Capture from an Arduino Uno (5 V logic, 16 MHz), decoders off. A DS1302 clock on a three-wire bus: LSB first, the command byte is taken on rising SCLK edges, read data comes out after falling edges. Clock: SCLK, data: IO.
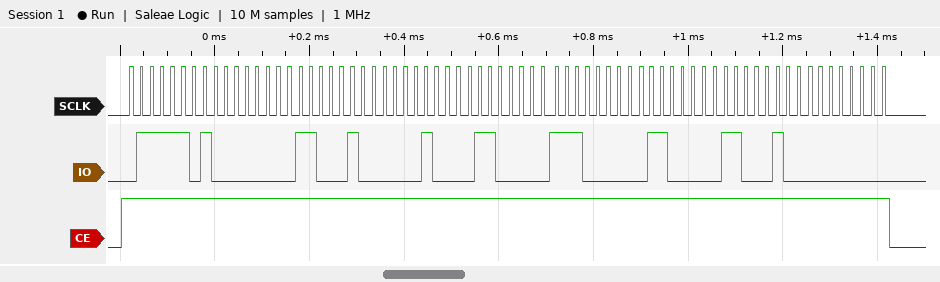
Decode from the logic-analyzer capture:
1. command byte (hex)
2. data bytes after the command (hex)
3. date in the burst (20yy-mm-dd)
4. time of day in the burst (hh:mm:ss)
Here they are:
0xBE
00 23 10 06 07 06 23 00
2023-07-06
10:23:00
